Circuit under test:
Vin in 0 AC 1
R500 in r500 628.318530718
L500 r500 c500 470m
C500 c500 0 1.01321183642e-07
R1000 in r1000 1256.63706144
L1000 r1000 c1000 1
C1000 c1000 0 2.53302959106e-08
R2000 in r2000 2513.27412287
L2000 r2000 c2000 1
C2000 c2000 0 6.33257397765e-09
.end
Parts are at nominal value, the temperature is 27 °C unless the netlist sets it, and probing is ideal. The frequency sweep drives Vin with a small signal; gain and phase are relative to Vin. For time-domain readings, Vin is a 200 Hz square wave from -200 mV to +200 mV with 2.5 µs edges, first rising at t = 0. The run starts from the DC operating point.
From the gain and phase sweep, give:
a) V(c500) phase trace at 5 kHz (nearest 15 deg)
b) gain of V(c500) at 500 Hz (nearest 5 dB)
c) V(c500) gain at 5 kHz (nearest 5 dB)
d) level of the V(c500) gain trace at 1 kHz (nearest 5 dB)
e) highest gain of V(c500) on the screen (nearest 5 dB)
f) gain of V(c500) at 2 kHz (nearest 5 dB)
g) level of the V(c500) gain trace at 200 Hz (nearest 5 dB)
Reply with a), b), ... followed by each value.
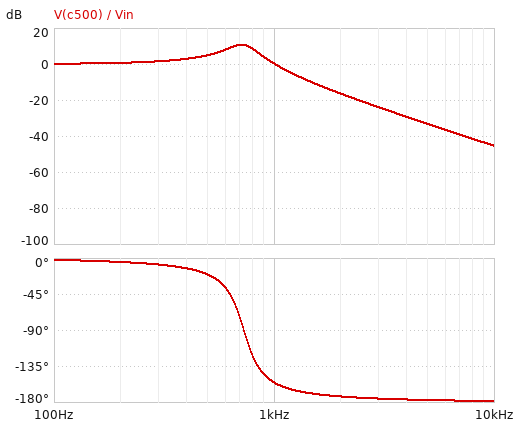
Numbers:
a) -180 deg
b) 5 dB
c) -35 dB
d) 0 dB
e) 10 dB
f) -15 dB
g) 0 dB
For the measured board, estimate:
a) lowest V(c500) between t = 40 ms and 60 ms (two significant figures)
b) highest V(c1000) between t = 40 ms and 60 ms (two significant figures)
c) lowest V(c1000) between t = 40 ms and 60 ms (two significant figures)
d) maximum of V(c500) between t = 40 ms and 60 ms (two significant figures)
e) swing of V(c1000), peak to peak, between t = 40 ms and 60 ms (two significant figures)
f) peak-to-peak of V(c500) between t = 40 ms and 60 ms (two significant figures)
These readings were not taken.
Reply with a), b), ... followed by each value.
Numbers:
a) -440 mV
b) 570 mV
c) -570 mV
d) 440 mV
e) 1.1 V
f) 880 mV
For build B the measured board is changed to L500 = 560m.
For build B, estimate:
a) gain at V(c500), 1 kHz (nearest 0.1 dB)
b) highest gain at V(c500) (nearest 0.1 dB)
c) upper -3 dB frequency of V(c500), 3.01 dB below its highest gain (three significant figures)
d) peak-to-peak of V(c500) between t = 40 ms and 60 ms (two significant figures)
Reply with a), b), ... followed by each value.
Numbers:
a) -2.3 dB
b) 11.5 dB
c) 741 Hz
d) 1.0 V
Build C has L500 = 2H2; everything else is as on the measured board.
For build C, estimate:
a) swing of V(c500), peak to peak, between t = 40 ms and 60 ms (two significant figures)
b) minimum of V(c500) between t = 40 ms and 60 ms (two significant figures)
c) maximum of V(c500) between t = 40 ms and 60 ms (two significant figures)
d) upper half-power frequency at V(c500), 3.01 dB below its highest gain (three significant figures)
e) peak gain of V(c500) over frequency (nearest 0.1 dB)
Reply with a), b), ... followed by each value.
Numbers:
a) 840 mV
b) -420 mV
c) 420 mV
d) 358 Hz
e) 17.4 dB
